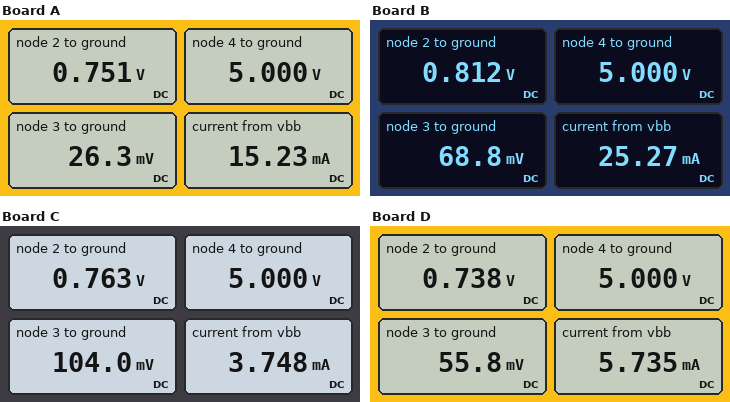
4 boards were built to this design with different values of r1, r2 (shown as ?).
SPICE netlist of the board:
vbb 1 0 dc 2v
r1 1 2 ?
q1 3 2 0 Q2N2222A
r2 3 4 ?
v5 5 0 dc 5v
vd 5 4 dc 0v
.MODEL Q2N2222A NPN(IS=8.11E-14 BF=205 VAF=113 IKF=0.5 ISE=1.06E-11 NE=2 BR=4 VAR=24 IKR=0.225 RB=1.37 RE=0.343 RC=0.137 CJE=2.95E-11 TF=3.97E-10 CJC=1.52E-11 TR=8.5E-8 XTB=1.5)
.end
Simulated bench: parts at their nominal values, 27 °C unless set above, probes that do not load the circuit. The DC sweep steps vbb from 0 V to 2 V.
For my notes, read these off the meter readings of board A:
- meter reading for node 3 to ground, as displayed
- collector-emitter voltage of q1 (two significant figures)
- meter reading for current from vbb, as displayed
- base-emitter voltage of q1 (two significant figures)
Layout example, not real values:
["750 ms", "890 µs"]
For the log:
["26.3 mV", "26 mV", "15.23 mA", "750 mV"]
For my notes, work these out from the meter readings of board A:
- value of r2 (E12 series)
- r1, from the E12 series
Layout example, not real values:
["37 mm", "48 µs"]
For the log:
["330 Ω", "82 Ω"]
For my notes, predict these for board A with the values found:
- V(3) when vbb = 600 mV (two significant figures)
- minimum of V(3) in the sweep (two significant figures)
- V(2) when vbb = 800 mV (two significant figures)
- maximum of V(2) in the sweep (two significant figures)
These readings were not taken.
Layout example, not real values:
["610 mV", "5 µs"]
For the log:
["4.7 V", "26 mV", "690 mV", "750 mV"]
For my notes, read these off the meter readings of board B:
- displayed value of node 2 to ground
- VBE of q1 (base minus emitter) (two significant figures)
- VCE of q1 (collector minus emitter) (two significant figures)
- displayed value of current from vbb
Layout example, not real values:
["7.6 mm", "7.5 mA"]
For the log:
["0.812 V", "810 mV", "69 mV", "25.27 mA"]
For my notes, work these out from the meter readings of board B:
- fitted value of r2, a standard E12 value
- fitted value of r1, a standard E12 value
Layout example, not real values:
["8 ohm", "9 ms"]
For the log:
["68 Ω", "47 Ω"]
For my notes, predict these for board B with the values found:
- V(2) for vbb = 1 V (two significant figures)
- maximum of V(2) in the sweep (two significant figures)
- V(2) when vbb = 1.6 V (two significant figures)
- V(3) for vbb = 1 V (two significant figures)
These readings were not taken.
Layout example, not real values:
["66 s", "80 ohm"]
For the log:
["760 mV", "810 mV", "790 mV", "85 mV"]
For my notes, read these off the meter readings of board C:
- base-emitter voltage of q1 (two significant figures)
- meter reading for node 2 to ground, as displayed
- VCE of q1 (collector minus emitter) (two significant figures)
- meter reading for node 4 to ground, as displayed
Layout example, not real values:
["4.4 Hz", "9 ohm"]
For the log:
["760 mV", "0.763 V", "100 mV", "5.000 V"]
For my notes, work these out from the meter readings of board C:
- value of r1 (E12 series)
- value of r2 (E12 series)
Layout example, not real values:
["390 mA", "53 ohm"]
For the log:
["330 Ω", "56 Ω"]
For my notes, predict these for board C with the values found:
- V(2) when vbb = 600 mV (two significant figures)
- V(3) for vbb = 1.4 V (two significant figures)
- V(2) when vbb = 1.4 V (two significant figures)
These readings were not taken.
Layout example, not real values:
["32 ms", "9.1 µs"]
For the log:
["600 mV", "120 mV", "760 mV"]
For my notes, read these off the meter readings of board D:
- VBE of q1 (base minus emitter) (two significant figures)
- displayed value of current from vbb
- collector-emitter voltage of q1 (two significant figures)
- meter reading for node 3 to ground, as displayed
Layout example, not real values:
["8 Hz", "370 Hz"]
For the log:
["740 mV", "5.735 mA", "56 mV", "55.8 mV"]
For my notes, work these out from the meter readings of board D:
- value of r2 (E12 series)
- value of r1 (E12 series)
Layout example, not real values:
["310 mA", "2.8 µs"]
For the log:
["120 Ω", "220 Ω"]
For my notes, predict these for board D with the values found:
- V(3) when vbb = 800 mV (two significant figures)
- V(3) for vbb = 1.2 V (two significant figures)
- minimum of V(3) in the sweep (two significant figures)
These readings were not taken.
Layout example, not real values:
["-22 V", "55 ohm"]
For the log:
["130 mV", "73 mV", "56 mV"]
